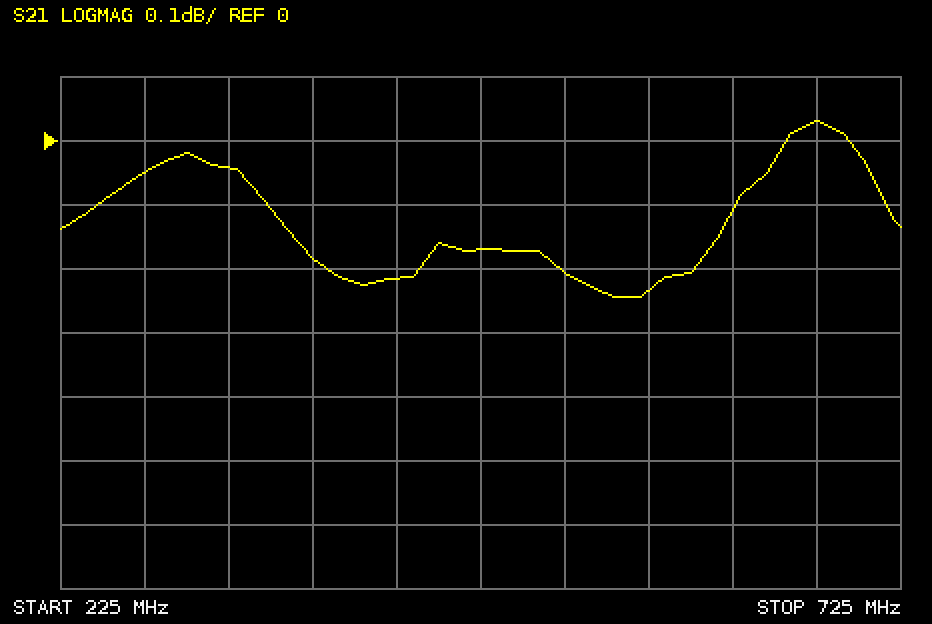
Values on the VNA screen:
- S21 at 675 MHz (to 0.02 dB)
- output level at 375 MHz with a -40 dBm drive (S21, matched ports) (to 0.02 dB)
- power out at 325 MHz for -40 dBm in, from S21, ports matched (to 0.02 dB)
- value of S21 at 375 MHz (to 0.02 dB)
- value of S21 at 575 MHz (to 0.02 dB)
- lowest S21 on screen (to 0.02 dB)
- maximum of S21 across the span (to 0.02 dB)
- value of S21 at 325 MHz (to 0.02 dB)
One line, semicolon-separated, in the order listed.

0.04 dB; -40.18 dBm; -40.04 dBm; -0.18 dB; -0.24 dB; -0.24 dB; 0.04 dB; -0.04 dB
